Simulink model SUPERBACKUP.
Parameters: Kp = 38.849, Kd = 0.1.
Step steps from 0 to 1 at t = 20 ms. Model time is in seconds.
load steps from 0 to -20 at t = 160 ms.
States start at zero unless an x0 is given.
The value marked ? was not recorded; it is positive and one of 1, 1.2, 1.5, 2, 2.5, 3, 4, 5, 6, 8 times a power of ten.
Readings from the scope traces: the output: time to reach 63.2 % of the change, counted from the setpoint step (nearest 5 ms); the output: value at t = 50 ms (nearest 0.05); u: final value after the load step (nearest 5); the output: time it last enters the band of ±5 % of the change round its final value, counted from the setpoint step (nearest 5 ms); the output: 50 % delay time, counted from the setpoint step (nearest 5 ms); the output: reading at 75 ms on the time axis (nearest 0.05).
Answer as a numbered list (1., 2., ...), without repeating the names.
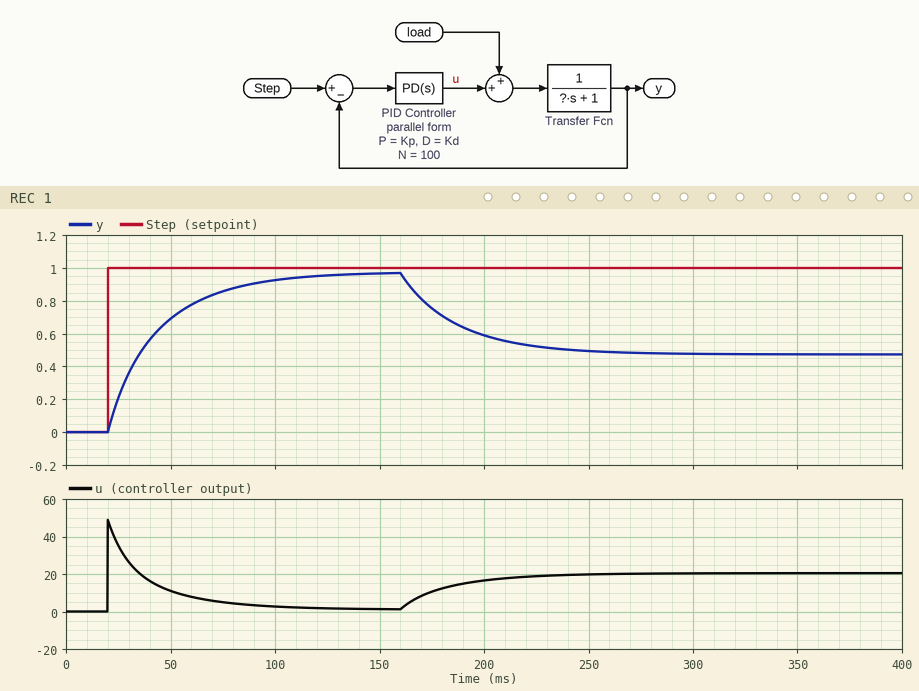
1. 25 ms
2. 0.70
3. 20
4. 80 ms
5. 15 ms
6. 0.85
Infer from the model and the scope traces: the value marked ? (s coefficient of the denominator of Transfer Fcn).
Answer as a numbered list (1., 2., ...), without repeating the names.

1. 1
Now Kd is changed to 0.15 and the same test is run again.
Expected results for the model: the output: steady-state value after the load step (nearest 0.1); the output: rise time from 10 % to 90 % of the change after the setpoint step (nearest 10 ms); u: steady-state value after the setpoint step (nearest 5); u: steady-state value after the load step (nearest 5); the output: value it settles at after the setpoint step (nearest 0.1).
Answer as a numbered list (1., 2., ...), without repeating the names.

1. 0.5
2. 60 ms
3. 0
4. 20
5. 1.0
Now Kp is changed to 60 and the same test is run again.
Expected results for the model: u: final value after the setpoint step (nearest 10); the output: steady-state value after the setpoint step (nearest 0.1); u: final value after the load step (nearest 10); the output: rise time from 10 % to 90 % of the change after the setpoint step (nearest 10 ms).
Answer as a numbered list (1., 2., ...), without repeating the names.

1. 0
2. 1.0
3. 20
4. 40 ms
